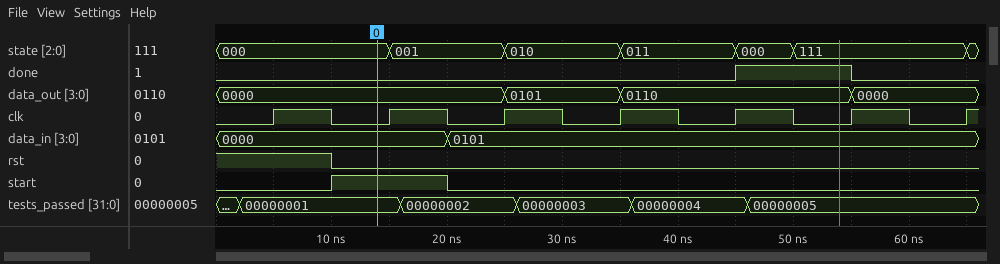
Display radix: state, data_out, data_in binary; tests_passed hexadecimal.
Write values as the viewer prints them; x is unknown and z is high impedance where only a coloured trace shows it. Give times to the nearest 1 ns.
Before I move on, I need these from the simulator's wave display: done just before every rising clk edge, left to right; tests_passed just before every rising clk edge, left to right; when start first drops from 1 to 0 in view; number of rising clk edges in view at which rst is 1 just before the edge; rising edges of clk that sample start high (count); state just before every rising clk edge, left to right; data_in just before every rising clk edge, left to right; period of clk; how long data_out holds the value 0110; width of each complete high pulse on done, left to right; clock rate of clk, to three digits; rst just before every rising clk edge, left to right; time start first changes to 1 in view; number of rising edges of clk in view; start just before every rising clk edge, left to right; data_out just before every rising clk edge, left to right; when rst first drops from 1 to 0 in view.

0 0 0 0 0 1 0
00000001, 00000001, 00000002, 00000003, 00000004, 00000005, 00000005
20 ns
1
1
000, 000, 001, 010, 011, 111, 111
0000, 0000, 0101, 0101, 0101, 0101, 0101
10 ns
20 ns
10 ns
100 MHz
1 0 0 0 0 0 0
10 ns
7
0 1 0 0 0 0 0
0000, 0000, 0000, 0101, 0110, 0110, 0000
10 ns
